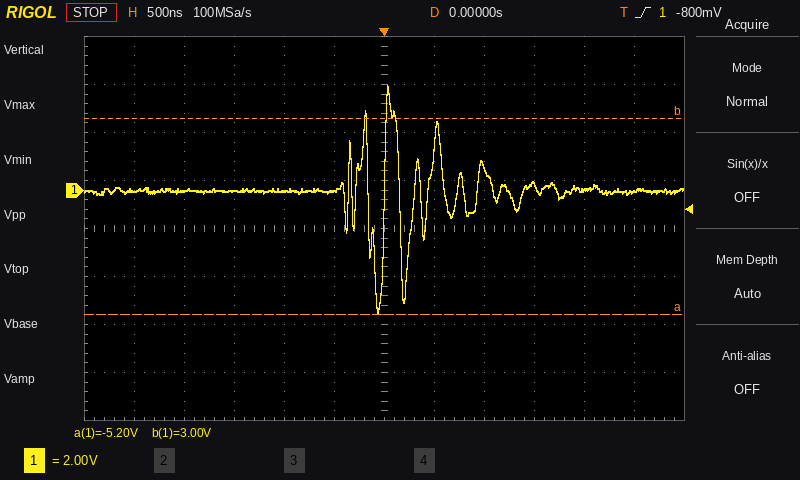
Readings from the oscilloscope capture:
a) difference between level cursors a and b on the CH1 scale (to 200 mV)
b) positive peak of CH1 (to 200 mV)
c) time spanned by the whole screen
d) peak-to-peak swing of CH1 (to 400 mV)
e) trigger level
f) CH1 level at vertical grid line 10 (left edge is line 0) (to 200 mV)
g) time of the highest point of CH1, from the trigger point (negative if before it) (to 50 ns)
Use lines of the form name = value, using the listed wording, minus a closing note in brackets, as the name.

difference between level cursors a and b on the CH1 scale = 8.2 V
positive peak of CH1 = 4.4 V
time spanned by the whole screen = 6 µs
peak-to-peak swing of CH1 = 9.6 V
trigger level = -800 mV
CH1 level at vertical grid line 10 (left edge is line 0) = 0.0 V
time of the highest point of CH1, from the trigger point (negative if before it) = +50 ns
